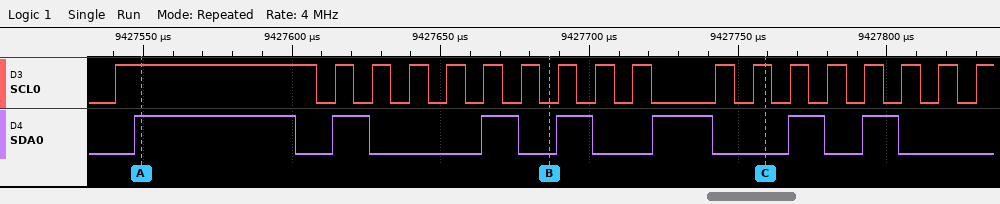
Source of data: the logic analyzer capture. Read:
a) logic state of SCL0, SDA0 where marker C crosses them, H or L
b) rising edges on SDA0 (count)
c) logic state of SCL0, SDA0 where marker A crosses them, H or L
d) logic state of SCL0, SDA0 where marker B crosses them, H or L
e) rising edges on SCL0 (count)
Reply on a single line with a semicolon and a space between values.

SCL0=H, SDA0=L; 7; SCL0=H, SDA0=H; SCL0=L, SDA0=L; 18
